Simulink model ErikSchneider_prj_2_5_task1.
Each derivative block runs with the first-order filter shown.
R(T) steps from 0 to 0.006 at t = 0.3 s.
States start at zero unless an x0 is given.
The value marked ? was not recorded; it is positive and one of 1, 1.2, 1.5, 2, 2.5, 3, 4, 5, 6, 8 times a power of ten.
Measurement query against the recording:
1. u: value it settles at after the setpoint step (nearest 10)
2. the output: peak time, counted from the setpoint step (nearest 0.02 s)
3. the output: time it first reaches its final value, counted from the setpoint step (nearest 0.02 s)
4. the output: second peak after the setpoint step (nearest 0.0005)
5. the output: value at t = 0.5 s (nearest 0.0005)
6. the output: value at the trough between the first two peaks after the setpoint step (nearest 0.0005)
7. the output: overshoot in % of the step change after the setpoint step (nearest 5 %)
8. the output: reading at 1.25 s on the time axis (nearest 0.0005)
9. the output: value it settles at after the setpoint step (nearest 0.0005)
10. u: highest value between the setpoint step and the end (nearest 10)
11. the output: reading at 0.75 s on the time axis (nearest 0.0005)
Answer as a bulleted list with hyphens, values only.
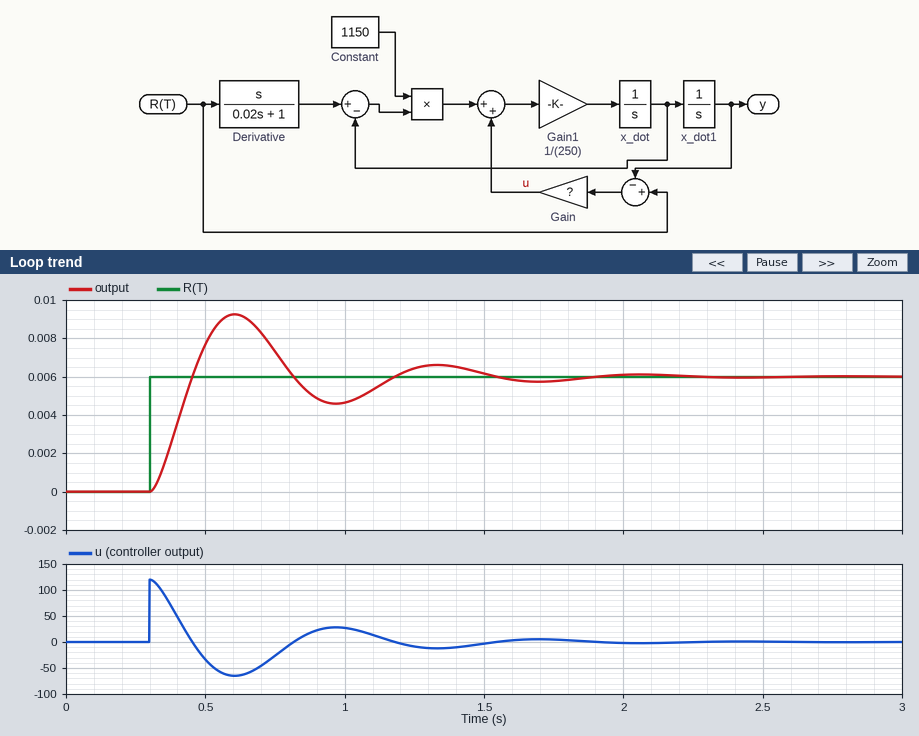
- 0
- 0.30 s
- 0.16 s
- 0.0065
- 0.0075
- 0.0045
- 55 %
- 0.0065
- 0.0060
- 120
- 0.0075
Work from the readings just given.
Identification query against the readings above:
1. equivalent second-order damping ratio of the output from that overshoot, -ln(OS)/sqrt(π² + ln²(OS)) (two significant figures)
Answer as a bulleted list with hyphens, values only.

- 0.19
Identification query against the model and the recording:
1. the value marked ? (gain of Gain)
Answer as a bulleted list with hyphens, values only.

- 20000
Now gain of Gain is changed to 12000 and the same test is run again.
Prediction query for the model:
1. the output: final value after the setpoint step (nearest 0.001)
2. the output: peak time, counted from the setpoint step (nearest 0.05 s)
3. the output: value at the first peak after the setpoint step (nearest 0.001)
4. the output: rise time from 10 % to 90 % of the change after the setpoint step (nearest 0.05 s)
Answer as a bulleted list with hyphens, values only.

- 0.006
- 0.40 s
- 0.009
- 0.15 s
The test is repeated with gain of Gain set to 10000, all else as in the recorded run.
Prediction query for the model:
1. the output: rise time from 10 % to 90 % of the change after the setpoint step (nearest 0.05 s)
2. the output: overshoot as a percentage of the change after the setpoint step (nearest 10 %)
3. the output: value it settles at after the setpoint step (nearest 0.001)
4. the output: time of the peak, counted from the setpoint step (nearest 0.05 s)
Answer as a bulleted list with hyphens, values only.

- 0.15 s
- 40 %
- 0.006
- 0.40 s
